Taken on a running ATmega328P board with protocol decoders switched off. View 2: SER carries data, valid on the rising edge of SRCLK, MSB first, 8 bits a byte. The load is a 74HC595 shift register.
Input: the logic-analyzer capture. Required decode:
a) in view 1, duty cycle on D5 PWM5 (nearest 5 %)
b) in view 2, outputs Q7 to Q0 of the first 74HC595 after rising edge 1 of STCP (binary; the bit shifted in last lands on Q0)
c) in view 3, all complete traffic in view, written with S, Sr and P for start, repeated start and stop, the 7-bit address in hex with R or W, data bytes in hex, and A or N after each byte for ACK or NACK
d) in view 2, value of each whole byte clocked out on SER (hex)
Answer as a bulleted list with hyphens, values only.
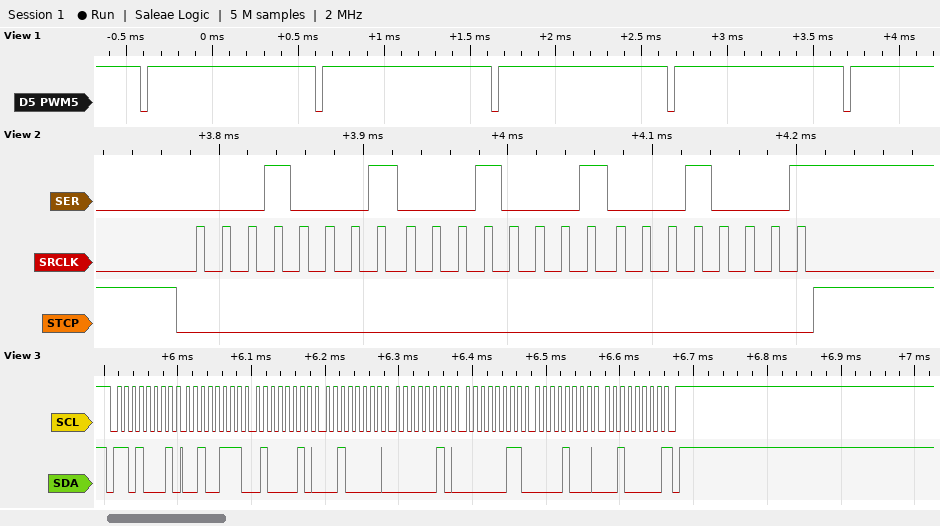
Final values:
- 95 %
- 00010001
- S 68R A 27 A 42 A 20 A 02 A 03 A 08 A 20 N P
- 11 11 11
